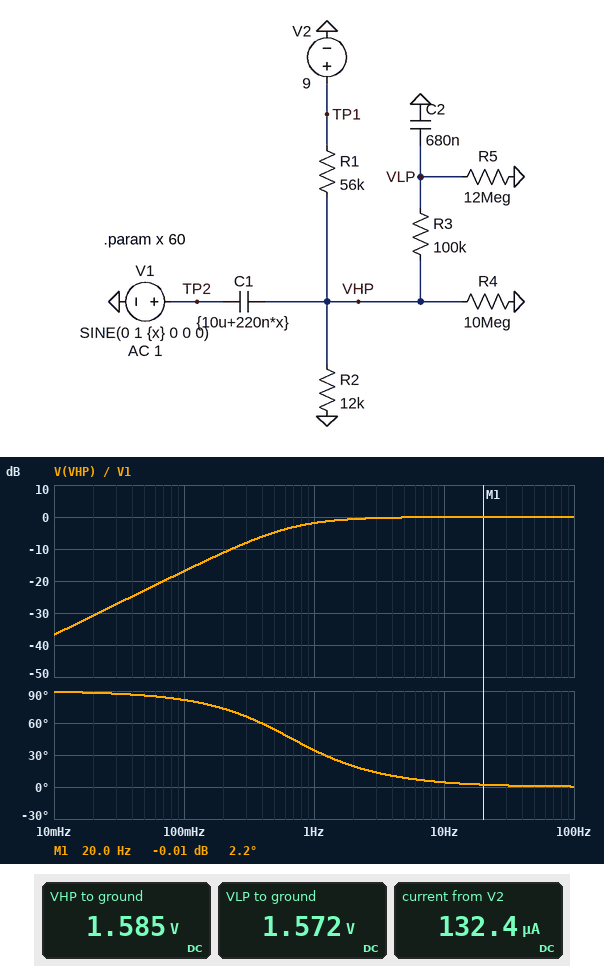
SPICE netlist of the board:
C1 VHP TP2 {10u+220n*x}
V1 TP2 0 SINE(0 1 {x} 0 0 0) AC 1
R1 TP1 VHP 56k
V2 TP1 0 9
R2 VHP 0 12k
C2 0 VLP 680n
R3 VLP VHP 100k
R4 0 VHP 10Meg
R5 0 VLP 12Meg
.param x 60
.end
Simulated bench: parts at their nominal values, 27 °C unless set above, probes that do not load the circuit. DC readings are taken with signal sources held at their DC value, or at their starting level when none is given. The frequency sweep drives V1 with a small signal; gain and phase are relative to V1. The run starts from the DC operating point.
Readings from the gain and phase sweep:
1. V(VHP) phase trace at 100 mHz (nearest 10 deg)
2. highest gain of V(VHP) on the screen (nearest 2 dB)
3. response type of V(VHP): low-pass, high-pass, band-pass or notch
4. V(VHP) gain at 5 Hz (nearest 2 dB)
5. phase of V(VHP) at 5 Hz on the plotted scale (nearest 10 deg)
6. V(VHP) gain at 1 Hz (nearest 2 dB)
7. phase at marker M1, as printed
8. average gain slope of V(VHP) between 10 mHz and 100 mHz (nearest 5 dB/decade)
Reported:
80 deg
0 dB
high-pass
0 dB
10 deg
-2 dB
2.2 deg
20 dB/decade
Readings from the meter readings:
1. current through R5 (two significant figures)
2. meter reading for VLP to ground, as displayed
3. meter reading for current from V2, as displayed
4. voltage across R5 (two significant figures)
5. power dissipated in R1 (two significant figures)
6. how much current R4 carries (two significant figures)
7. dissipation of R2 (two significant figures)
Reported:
130 nA
1.572 V
132.4 µA
1.6 V
980 µW
160 nA
210 µW
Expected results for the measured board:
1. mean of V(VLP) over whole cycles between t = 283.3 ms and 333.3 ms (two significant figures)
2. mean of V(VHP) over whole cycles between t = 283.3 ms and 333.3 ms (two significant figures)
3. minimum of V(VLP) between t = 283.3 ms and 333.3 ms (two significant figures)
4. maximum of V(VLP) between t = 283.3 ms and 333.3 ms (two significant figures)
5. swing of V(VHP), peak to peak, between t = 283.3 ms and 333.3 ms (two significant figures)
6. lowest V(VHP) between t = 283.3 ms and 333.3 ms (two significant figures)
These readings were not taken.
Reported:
1.6 V
1.6 V
1.5 V
1.6 V
2.0 V
580 mV
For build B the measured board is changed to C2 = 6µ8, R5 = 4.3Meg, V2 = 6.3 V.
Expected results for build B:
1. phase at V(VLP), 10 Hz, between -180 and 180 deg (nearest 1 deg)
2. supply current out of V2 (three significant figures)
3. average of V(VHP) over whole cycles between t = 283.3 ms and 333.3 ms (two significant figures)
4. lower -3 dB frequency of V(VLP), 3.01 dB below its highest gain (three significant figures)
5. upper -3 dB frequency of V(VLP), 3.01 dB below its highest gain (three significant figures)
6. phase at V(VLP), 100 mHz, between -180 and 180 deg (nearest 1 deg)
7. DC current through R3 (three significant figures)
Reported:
-84 deg
92.7 µA
1.1 V
145 mHz
1.15 Hz
57 deg
252 nA
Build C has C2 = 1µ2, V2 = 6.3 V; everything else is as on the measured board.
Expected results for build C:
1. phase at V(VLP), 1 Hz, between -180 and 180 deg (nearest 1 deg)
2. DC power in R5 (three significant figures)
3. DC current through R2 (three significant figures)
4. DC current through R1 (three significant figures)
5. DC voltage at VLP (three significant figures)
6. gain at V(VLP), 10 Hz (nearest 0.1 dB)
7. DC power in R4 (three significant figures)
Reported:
-2 deg
101 nW
92.5 µA
92.7 µA
1.10 V
-17.7 dB
123 nW
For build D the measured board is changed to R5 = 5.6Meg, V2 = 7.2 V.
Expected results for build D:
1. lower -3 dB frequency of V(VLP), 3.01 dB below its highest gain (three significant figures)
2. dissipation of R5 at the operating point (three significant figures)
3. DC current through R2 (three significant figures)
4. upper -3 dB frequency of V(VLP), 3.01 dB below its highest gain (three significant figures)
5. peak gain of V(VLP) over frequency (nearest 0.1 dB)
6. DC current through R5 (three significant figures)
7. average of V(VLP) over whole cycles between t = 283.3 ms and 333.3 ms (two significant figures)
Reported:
460 mHz
277 nW
106 µA
3.61 Hz
-2.6 dB
222 nA
1.2 V
